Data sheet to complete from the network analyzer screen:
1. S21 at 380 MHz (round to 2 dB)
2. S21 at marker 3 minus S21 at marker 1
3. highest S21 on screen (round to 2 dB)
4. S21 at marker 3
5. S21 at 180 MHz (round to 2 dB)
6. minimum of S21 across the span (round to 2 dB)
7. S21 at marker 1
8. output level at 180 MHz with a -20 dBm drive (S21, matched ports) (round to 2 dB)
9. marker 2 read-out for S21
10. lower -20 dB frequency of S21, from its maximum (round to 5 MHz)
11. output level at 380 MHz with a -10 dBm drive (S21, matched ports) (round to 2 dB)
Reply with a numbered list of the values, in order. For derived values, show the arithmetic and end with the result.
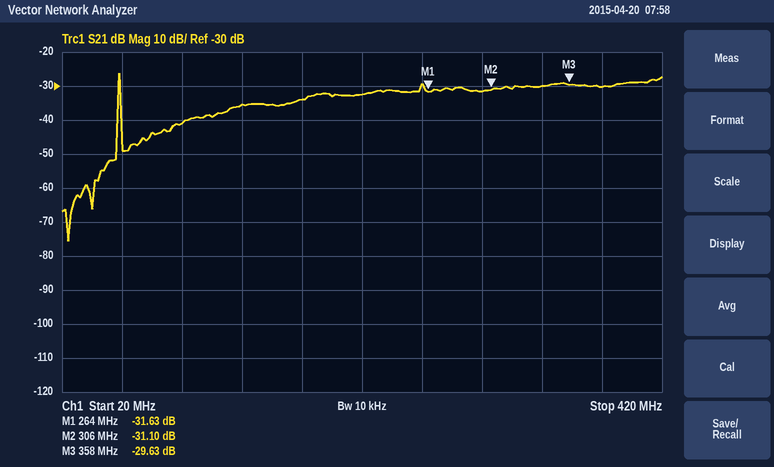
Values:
1. -30 dB
2. -29.63 − (-31.63) = 2.00 dB
3. -26 dB
4. -29.63 dB
5. -34 dB
6. -76 dB
7. -31.63 dB
8. -20 dBm + (-34 dB) = -54 dBm
9. -31.10 dB
10. 55 MHz
11. -10 dBm + (-30 dB) = -40 dBm
